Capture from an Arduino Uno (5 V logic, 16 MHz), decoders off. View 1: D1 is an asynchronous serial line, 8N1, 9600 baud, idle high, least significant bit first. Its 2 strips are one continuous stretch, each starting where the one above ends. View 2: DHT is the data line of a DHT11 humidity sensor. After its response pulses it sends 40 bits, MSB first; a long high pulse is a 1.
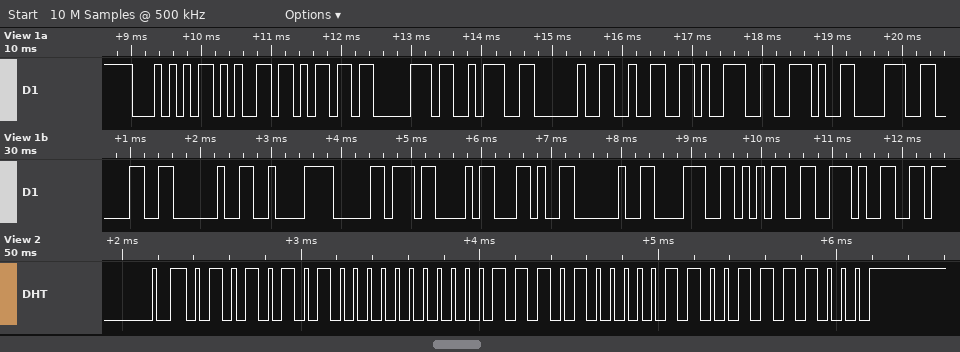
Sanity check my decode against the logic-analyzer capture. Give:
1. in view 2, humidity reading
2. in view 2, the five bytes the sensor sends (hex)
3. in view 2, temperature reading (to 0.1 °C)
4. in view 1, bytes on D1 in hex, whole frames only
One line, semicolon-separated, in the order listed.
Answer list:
85 %; 55 00 1D 06 78; 29.6 °C; 54 65 6D 70 3A 20 32 39 2E 38 30 20 C2 B0 43 2C 20 38 35 2E
